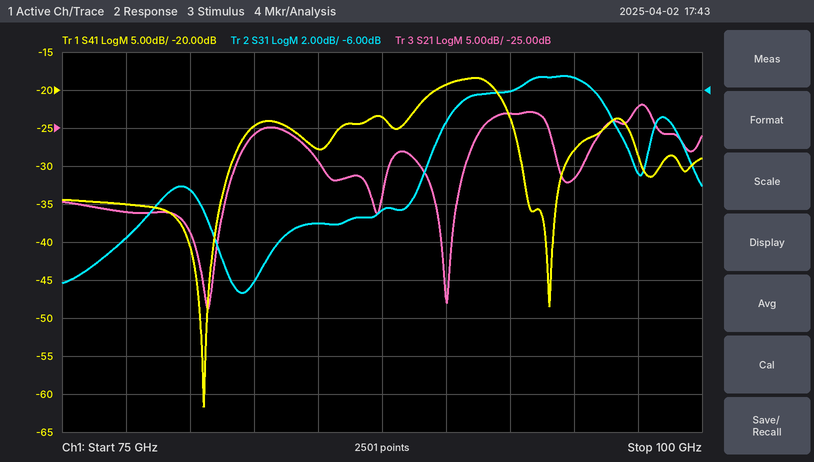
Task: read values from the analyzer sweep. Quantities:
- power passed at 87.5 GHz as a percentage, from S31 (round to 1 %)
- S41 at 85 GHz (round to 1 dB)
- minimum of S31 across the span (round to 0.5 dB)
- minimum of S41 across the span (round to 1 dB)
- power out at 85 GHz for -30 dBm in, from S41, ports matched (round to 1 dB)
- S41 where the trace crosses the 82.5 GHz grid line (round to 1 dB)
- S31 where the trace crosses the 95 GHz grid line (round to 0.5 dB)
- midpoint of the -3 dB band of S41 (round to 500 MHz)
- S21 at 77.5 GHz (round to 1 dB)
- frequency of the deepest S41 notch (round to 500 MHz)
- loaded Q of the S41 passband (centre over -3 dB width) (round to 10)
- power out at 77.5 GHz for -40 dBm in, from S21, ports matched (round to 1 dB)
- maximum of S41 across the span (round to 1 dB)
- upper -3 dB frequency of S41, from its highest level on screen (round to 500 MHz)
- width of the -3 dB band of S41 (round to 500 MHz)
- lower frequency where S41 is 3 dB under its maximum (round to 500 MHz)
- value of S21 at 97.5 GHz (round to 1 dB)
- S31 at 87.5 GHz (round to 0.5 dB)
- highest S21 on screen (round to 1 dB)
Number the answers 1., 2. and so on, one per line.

1. 6 %
2. -28 dB
3. -16.5 dB
4. -62 dB
5. -58 dBm
6. -25 dB
7. -5.5 dB
8. 90.5 GHz
9. -36 dB
10. 80.5 GHz
11. 30
12. -76 dBm
13. -18 dB
14. 92.0 GHz
15. 3.0 GHz
16. 89.0 GHz
17. -22 dB
18. -12.5 dB
19. -22 dB
